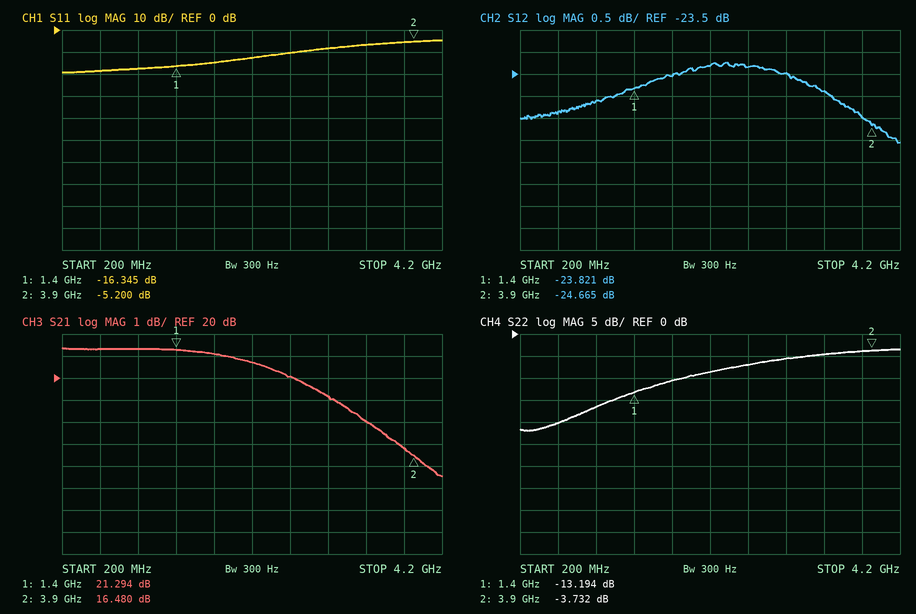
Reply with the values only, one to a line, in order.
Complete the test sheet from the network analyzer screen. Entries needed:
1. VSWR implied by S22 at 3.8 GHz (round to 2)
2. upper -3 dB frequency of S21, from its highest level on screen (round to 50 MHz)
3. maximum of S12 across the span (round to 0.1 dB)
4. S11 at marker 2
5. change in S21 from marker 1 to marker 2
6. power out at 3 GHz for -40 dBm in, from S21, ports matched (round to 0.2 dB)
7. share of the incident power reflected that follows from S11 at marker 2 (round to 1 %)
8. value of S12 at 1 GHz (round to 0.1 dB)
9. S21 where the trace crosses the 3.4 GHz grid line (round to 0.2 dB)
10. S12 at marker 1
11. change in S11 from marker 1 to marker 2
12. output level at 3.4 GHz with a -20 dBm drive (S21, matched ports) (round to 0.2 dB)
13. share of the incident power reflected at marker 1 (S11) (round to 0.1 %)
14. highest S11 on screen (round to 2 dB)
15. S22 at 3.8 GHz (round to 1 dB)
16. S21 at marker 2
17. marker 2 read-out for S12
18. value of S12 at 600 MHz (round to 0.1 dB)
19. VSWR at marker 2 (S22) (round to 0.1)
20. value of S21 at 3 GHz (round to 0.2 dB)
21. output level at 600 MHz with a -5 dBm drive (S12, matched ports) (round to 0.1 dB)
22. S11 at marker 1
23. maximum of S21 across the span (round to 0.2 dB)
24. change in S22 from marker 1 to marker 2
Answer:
4
3.30 GHz
-23.2 dB
-5.200 dB
-4.814 dB
-20.8 dBm
30 %
-24.1 dB
18.0 dB
-23.821 dB
11.145 dB
-2.0 dBm
2.3 %
-4 dB
-4 dB
16.480 dB
-24.665 dB
-24.4 dB
4.7
19.2 dB
-29.4 dBm
-16.345 dB
21.4 dB
9.462 dB
